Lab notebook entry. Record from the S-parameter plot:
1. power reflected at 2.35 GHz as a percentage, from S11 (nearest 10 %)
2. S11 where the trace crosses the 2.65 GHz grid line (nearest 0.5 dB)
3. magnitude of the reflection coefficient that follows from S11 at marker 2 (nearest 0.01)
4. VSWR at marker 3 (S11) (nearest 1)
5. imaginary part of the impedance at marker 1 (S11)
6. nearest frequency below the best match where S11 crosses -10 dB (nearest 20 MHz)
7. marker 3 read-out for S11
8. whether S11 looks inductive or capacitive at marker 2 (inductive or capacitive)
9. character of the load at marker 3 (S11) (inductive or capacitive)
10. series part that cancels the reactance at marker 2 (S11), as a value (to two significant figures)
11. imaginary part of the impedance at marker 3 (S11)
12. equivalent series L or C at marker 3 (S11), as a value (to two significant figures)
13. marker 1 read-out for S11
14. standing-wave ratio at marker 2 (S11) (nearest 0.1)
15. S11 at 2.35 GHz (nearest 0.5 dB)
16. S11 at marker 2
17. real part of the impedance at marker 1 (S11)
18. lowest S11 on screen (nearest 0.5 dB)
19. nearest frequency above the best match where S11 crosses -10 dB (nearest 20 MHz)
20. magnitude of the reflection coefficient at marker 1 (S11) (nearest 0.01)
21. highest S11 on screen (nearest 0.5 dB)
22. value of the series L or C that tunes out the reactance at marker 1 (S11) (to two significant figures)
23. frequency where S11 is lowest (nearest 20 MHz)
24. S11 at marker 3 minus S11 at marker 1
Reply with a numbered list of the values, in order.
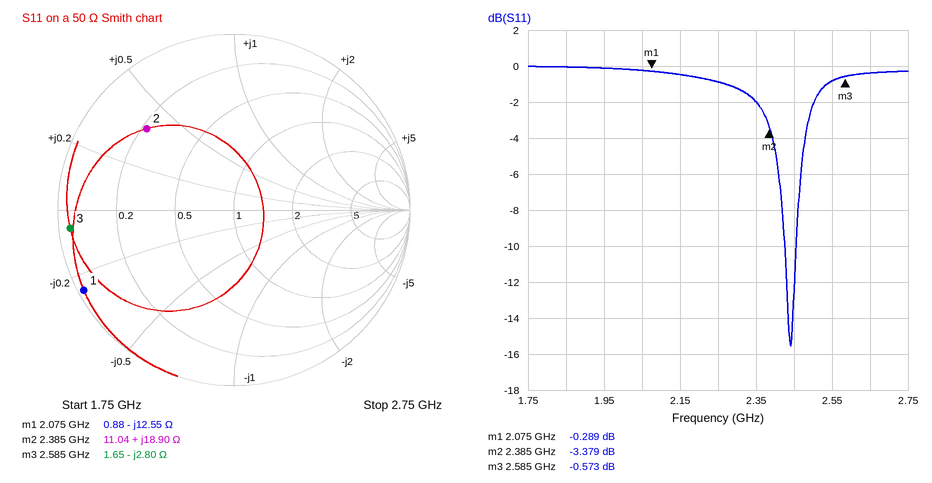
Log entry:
1. 60 %
2. -0.5 dB
3. 0.68
4. 30
5. -12.55 Ω
6. 2.42 GHz
7. -0.573 dB
8. inductive
9. capacitive
10. 3.5 pF
11. -2.80 Ω
12. 22 pF
13. -0.289 dB
14. 5.2
15. -2.0 dB
16. -3.379 dB
17. 0.88 Ω
18. -15.5 dB
19. 2.46 GHz
20. 0.97
21. 0.0 dB
22. 960 pH
23. 2.44 GHz
24. -0.284 dB
